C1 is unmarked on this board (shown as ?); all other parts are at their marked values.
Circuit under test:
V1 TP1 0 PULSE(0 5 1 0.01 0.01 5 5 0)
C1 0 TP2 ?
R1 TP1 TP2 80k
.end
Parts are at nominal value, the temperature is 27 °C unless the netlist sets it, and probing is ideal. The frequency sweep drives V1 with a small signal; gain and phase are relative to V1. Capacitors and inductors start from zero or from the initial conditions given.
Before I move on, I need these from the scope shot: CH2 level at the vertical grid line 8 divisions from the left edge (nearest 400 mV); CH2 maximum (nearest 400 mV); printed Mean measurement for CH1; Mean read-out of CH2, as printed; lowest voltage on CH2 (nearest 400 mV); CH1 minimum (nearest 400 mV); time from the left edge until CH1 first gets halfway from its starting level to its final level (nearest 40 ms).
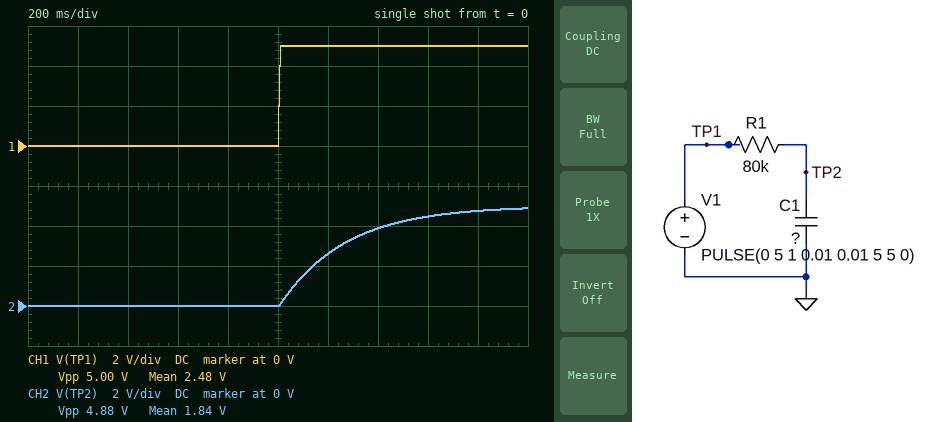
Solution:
4.4 V
4.8 V
2.48 V
1.84 V
0 V
0 V
1.00 s
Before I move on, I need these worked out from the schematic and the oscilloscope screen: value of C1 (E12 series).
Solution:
3.3 µF
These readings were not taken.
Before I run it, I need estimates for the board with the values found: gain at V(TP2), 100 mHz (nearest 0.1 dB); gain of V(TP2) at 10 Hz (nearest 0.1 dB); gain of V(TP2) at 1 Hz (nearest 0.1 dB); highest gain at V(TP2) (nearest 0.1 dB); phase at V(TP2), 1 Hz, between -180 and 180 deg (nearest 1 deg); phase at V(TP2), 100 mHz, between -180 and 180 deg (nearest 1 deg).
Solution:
-0.1 dB
-24.4 dB
-5.7 dB
0 dB
-59 deg
-9 deg
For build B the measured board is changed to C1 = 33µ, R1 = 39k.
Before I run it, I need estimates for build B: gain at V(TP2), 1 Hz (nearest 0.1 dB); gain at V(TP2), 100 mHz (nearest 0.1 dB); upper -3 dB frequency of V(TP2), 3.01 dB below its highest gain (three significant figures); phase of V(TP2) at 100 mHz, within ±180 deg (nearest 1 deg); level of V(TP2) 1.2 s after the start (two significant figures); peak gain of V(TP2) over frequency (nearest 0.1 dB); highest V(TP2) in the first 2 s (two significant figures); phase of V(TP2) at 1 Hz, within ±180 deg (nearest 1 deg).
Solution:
-18.2 dB
-2.2 dB
124 mHz
-39 deg
700 mV
0 dB
2.7 V
-83 deg
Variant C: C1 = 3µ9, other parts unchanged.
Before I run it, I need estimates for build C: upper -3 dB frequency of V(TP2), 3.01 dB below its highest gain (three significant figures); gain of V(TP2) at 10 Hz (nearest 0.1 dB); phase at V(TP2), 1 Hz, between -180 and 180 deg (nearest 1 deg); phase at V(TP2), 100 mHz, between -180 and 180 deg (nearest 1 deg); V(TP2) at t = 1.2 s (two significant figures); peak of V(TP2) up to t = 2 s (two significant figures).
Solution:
510 mHz
-25.9 dB
-63 deg
-11 deg
2.3 V
4.8 V
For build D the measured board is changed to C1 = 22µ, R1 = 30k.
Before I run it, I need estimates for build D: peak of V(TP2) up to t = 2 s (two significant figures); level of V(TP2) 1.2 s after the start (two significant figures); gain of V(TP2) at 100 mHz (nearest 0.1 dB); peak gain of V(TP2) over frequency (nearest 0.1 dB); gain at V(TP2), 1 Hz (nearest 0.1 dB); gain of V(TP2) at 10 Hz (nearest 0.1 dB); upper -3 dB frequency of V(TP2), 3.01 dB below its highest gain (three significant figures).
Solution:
3.9 V
1.3 V
-0.7 dB
0 dB
-12.6 dB
-32.4 dB
241 mHz
